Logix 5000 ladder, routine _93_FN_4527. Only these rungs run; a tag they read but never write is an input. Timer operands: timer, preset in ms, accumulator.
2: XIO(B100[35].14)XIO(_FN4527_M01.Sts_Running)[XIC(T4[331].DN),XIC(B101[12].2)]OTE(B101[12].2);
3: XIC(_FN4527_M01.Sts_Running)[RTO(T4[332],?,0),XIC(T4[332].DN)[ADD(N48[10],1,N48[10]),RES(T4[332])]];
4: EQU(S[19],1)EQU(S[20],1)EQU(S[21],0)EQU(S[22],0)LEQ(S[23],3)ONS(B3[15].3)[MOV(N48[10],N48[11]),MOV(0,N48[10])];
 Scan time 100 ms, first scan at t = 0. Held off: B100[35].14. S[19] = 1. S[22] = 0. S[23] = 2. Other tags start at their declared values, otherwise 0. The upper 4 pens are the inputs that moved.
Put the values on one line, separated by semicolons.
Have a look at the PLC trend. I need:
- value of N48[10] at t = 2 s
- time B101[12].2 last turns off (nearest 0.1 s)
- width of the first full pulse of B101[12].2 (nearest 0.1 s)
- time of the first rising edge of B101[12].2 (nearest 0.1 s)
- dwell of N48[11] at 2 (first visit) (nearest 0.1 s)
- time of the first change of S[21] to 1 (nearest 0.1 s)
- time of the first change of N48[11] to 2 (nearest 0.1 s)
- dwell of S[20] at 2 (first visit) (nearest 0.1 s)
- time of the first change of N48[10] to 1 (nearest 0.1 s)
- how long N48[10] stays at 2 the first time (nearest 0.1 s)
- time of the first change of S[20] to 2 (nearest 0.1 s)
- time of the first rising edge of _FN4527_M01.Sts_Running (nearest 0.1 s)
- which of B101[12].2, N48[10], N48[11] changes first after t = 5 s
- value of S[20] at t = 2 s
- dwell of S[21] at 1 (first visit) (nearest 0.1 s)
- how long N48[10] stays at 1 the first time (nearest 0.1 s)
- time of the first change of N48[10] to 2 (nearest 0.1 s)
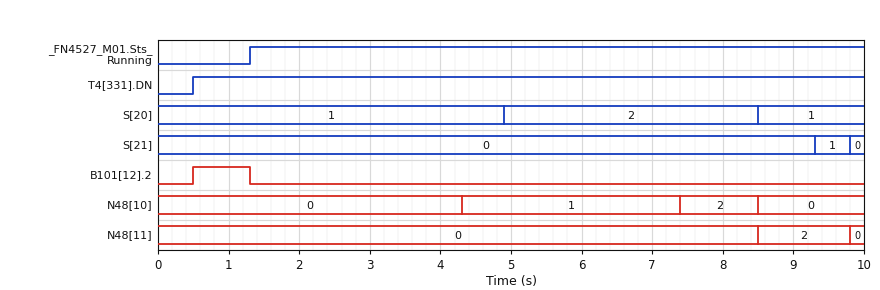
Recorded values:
0; 1.3 s; 0.8 s; 0.5 s; 1.3 s; 9.3 s; 8.5 s; 3.6 s; 4.3 s; 1.1 s; 4.9 s; 1.3 s; N48[10]; 1; 0.5 s; 3.1 s; 7.4 s
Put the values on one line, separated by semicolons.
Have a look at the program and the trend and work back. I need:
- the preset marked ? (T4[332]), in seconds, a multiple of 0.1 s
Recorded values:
3.0 s
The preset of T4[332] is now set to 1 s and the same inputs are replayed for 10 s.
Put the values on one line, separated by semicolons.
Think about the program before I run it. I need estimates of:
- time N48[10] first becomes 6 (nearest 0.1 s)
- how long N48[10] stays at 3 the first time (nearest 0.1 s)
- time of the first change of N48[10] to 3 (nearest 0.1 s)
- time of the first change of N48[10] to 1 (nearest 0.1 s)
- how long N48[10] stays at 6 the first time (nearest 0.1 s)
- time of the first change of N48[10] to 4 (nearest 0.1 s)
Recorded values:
7.8 s; 1.1 s; 4.5 s; 2.3 s; 0.7 s; 5.6 s
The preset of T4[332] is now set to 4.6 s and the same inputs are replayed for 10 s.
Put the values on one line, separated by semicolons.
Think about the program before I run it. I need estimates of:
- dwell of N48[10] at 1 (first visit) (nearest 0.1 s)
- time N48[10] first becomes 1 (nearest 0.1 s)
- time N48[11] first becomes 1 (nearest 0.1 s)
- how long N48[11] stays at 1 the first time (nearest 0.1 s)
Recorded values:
2.6 s; 5.9 s; 8.5 s; 1.3 s
